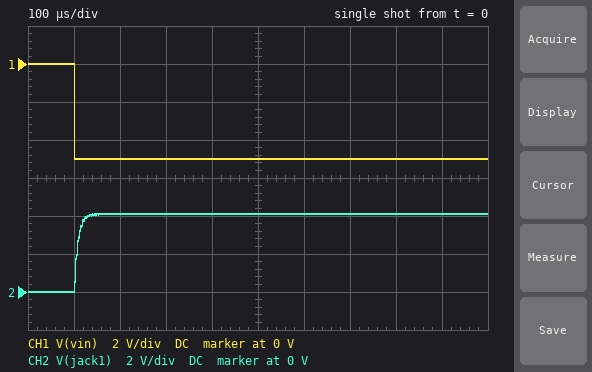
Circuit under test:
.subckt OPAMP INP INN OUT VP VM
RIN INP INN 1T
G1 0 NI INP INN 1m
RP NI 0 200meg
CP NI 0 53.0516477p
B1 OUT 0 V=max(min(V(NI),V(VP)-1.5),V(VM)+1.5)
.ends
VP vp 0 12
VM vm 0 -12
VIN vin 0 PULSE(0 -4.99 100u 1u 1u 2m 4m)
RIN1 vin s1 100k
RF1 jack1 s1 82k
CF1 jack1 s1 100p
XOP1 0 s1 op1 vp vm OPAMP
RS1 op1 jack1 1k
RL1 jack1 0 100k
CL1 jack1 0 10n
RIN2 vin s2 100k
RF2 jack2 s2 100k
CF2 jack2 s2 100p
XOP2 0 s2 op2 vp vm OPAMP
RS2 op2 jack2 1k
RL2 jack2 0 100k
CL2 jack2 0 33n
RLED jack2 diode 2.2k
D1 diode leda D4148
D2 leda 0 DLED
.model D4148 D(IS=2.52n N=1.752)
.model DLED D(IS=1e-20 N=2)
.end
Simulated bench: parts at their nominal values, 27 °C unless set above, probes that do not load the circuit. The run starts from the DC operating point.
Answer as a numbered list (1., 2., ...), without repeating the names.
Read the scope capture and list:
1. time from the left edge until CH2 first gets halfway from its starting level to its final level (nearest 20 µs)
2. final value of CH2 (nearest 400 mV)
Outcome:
1. 100 µs
2. 4.0 V
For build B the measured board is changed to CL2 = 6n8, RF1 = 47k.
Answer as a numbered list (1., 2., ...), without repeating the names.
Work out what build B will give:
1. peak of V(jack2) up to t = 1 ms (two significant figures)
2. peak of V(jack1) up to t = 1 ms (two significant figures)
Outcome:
1. 5.0 V
2. 2.4 V
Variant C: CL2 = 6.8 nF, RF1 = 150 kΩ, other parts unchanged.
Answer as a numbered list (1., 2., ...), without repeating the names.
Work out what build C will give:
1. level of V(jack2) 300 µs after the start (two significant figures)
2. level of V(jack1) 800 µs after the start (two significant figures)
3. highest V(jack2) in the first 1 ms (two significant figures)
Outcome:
1. 5.0 V
2. 7.5 V
3. 5.0 V
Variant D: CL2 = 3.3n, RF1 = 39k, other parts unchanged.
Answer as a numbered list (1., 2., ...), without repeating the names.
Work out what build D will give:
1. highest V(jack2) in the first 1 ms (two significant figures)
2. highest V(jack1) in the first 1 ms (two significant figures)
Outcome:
1. 5.0 V
2. 2.0 V
